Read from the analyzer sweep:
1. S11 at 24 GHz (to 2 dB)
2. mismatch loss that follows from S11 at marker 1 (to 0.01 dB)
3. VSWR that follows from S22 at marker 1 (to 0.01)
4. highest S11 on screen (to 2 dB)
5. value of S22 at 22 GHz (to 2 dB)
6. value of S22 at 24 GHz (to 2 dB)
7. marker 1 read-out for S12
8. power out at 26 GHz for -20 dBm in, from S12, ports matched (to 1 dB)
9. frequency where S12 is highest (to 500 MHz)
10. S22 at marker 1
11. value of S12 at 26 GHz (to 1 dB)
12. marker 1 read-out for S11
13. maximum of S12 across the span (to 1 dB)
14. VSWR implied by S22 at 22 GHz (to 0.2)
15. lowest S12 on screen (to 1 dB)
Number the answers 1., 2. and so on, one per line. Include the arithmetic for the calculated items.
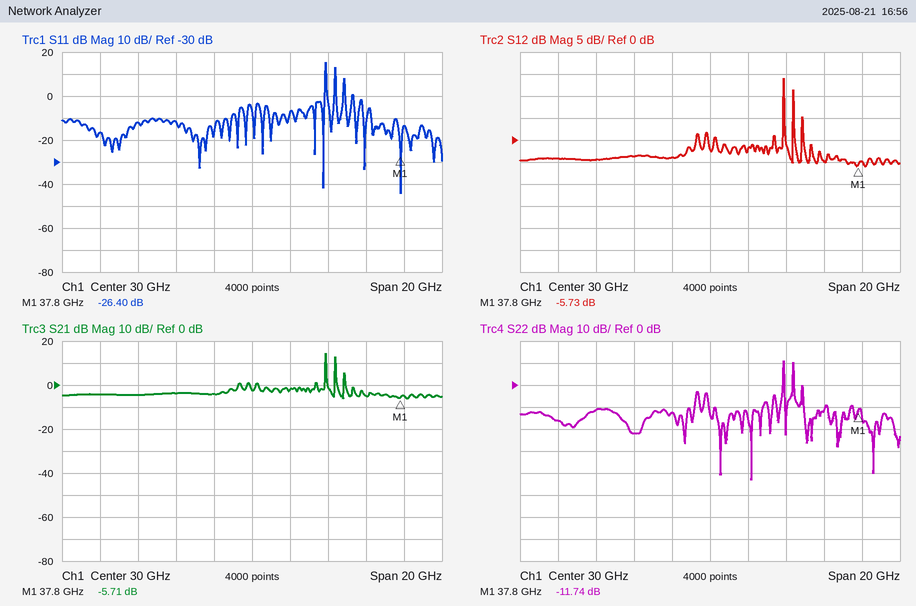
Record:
1. -12 dB
2. −10 log10(1 − 10^(-26.4/10)) ≈ 0.01 dB
3. (1 + 0.2588)/(1 − 0.2588) ≈ 1.70
4. 16 dB
5. -16 dB
6. -12 dB
7. -5.73 dB
8. -20 dBm + (-4 dB) = -24 dBm
9. 34.0 GHz
10. -11.74 dB
11. -4 dB
12. -26.40 dB
13. 14 dB
14. |Γ| = 10^(-16/20) = 0.1585; VSWR = (1 + 0.1585)/(1 − 0.1585) ≈ 1.4
15. -6 dB
